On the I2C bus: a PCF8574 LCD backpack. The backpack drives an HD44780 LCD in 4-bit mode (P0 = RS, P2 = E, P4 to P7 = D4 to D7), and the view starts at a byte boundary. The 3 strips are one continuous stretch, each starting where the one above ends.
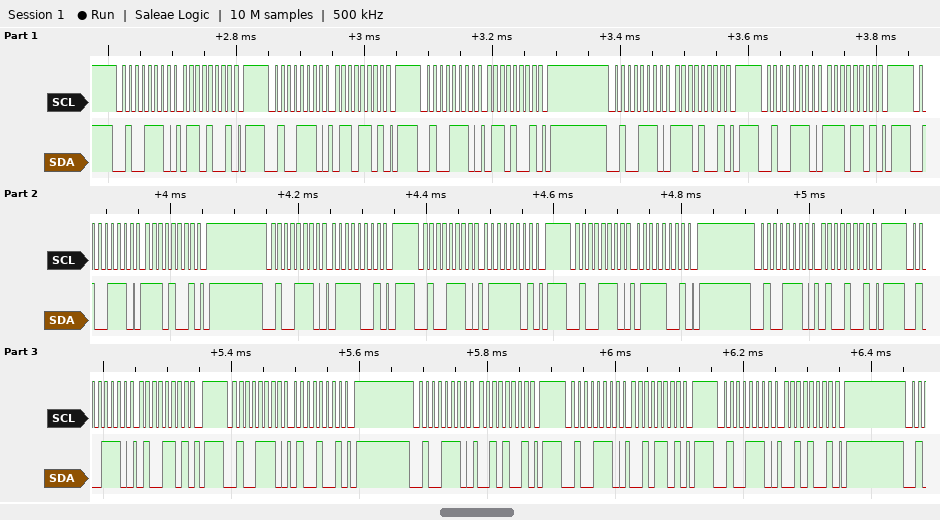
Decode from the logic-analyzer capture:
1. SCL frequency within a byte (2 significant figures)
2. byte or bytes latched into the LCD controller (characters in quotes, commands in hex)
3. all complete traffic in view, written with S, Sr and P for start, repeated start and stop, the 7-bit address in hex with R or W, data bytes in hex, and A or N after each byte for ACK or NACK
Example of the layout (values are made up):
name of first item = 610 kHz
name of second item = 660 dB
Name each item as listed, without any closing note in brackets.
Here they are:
SCL frequency within a byte = 100 kHz
byte or bytes latched into the LCD controller = 'n' 't'
all complete traffic in view, written with S, Sr and P for start, repeated start and stop, the 7-bit address in hex with R or W, data bytes in hex, and A or N after each byte for ACK or NACK = S 27W A 69 A P S 27W A 6D A P S 27W A 69 A P S 27W A E9 A P S 27W A ED A P S 27W A E9 A P S 27W A 79 A P S 27W A 7D A P S 27W A 79 A P S 27W A 49 A P S 27W A 4D A P S 27W A 49 A P S 27W A 29 A P S 27W A 2D A P S 27W A 29 A P
